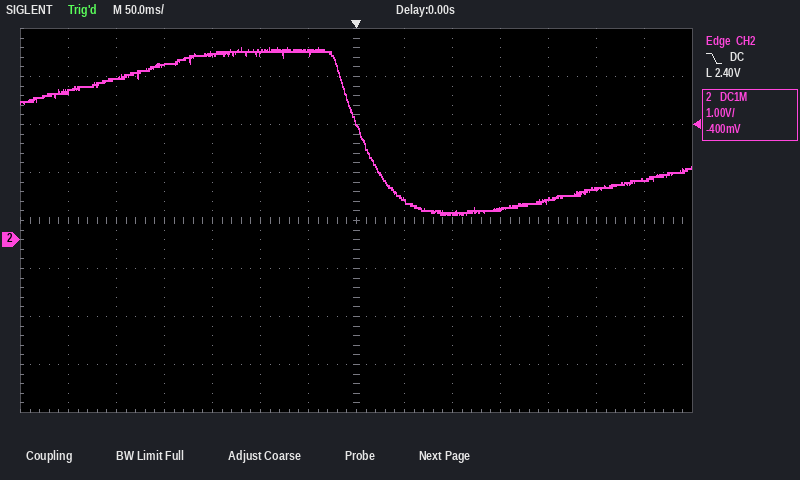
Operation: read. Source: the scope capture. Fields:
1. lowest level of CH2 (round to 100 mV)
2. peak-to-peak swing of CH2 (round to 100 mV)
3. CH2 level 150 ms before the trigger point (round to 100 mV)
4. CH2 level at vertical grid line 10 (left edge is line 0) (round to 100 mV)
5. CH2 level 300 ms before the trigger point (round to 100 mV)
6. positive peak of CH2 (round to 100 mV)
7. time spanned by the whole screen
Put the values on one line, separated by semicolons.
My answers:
500 mV; 3.5 V; 3.9 V; 600 mV; 3.1 V; 4.0 V; 700 ms
